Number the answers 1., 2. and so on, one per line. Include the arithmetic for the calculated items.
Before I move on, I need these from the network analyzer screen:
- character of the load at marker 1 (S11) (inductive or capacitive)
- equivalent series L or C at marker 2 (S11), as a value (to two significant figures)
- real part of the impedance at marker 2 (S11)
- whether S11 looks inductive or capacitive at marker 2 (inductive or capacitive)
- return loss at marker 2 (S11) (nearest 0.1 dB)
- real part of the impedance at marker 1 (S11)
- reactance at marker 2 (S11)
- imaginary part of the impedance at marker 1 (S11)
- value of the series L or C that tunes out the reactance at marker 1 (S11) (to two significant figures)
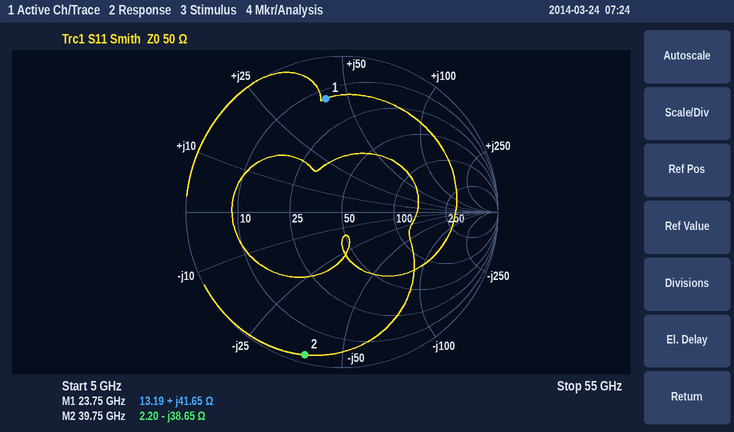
1. inductive
2. C = 1/(2π × 39.75 GHz × 38.65 Ω) ≈ 104 fF, so 100 fF to two significant figures
3. 2.20 Ω
4. capacitive
5. 0.5 dB
6. 13.19 Ω
7. -38.65 Ω
8. +41.65 Ω
9. C = 1/(2π × 23.75 GHz × 41.65 Ω) ≈ 161 fF, so 160 fF to two significant figures
